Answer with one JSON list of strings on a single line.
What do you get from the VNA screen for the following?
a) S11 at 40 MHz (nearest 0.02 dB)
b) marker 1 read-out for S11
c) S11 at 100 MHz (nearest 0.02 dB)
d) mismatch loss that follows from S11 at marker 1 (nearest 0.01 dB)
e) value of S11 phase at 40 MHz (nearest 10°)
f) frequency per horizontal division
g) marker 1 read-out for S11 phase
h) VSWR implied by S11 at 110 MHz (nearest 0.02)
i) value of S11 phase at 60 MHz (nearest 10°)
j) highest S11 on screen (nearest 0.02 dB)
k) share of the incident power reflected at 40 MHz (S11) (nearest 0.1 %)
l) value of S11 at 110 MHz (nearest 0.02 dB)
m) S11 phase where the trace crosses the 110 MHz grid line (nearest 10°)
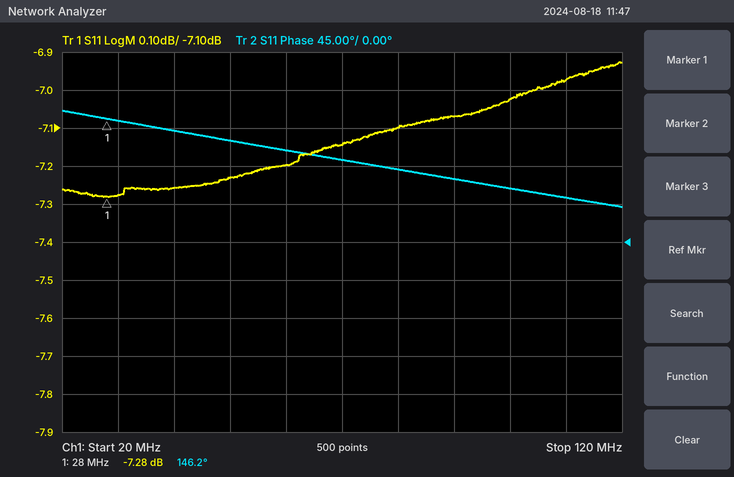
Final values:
["-7.26 dB", "-7.28 dB", "-7.02 dB", "0.90 dB", "130°", "10 MHz", "146.2°", "2.62", "110°", "-6.92 dB", "18.8 %", "-6.98 dB", "50°"]
